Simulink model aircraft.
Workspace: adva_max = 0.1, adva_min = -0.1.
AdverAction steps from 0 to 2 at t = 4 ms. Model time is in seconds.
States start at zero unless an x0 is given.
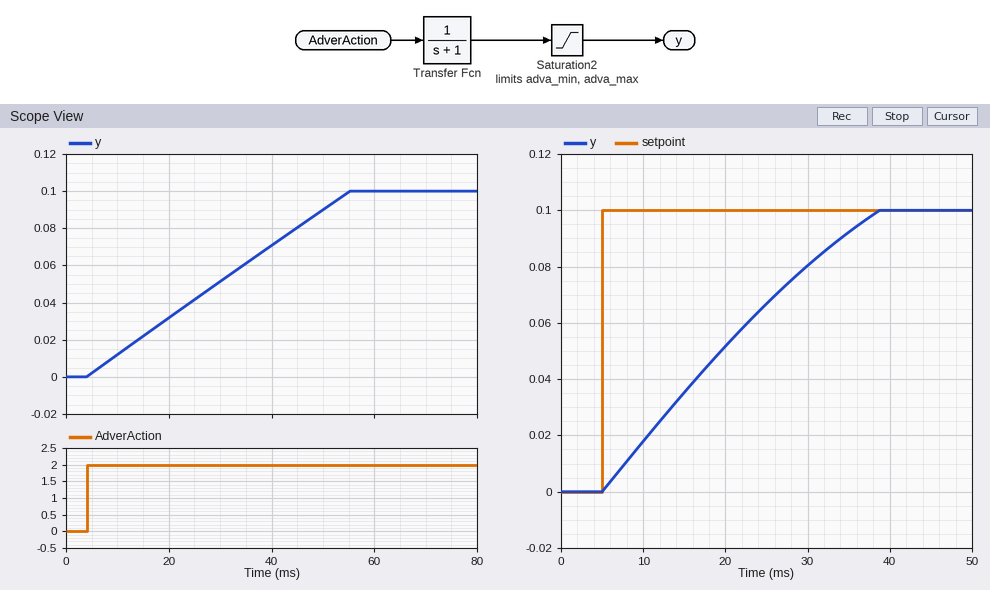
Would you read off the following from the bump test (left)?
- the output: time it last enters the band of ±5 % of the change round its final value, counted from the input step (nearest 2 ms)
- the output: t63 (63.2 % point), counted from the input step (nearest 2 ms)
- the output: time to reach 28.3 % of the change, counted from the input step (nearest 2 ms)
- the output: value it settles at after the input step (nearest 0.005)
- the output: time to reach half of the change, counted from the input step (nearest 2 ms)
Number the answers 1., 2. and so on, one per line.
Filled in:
1. 48 ms
2. 32 ms
3. 14 ms
4. 0.100
5. 26 ms
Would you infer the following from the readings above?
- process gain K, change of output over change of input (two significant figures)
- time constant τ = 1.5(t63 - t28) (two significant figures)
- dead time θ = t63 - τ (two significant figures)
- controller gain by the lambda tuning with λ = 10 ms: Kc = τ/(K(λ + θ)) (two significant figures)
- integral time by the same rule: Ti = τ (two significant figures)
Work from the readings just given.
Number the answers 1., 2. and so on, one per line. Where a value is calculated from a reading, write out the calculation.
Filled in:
1. (0.1 - 0) / 2 = 0.050
2. 1.5 × (32 - 14) = 27 ms
3. 32 - 27 = 5.0 ms
4. 27 / (0.05 × (10 + 5)) = 36
5. 27 ms
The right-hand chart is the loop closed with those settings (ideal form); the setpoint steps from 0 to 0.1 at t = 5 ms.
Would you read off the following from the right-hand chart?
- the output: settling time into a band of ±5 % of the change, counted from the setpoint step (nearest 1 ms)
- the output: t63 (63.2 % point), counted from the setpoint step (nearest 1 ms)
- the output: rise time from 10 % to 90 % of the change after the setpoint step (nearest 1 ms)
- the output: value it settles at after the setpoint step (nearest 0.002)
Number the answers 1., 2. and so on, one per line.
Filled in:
1. 31 ms
2. 19 ms
3. 26 ms
4. 0.100
